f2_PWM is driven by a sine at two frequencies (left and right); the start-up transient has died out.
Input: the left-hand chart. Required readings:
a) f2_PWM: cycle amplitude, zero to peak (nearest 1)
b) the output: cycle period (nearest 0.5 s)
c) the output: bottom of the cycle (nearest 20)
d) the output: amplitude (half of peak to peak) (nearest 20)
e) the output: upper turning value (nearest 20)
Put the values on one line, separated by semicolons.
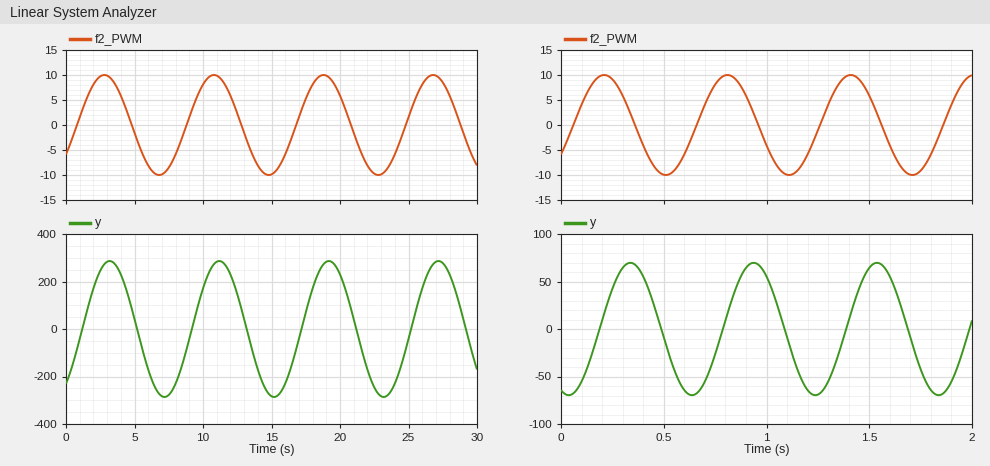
10; 8.0 s; -280; 280; 280
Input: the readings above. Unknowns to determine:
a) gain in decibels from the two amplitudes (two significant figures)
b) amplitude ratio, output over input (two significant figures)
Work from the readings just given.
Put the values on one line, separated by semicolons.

29 dB; 28
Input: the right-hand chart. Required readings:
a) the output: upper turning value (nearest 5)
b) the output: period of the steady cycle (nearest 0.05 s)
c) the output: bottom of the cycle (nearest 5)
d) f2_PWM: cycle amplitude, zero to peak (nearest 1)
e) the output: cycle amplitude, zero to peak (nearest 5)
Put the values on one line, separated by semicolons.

70; 0.60 s; -70; 10; 70
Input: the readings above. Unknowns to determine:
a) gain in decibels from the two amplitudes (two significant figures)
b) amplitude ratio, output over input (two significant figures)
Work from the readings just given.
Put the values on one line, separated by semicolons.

17 dB; 7.0
